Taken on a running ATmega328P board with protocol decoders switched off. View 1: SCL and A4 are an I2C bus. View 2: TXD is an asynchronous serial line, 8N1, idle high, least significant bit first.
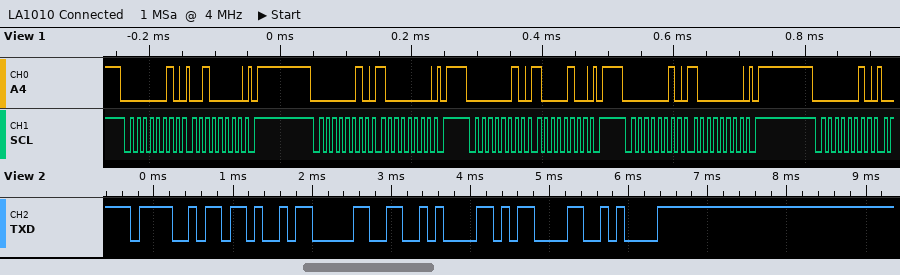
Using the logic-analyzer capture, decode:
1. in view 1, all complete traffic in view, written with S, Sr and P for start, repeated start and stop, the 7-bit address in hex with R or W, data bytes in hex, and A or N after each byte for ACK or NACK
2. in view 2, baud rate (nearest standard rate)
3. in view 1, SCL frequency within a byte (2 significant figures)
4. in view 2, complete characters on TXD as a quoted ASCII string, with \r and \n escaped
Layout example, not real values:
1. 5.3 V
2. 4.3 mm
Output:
1. S 01W A 20 A P S 01W A 80 A P S 01W A 84 A P S 01W A 80 A P S 01W A
2. 9600 baud
3. 100 kHz
4. "OK0\n\r\n"
